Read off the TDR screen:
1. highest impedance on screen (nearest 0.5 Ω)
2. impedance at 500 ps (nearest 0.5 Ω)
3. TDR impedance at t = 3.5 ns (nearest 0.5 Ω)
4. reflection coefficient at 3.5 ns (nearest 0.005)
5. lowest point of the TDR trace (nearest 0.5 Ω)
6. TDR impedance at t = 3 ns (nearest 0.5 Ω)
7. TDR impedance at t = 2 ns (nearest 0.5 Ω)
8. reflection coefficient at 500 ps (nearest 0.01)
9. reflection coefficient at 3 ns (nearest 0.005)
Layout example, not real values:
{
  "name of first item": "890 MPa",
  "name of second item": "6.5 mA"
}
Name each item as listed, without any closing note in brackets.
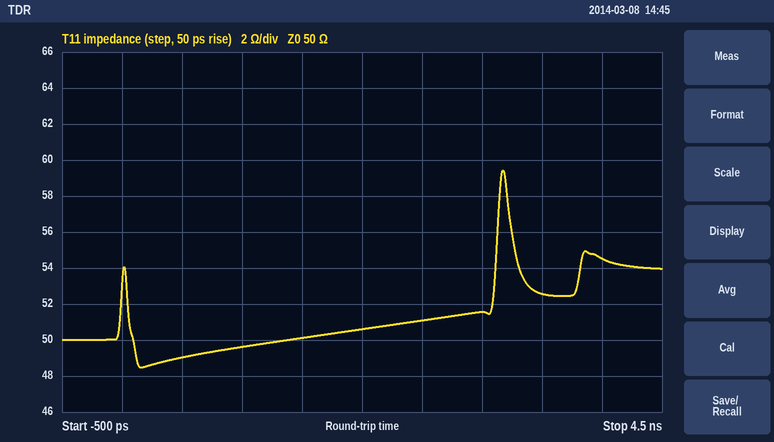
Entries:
{
  "highest impedance on screen": "59.5 Ω",
  "impedance at 500 ps": "49.0 Ω",
  "TDR impedance at t = 3.5 ns": "52.5 Ω",
  "reflection coefficient at 3.5 ns": "+0.025",
  "lowest point of the TDR trace": "48.5 Ω",
  "TDR impedance at t = 3 ns": "51.5 Ω",
  "TDR impedance at t = 2 ns": "50.5 Ω",
  "reflection coefficient at 500 ps": "-0.01",
  "reflection coefficient at 3 ns": "+0.015"
}
